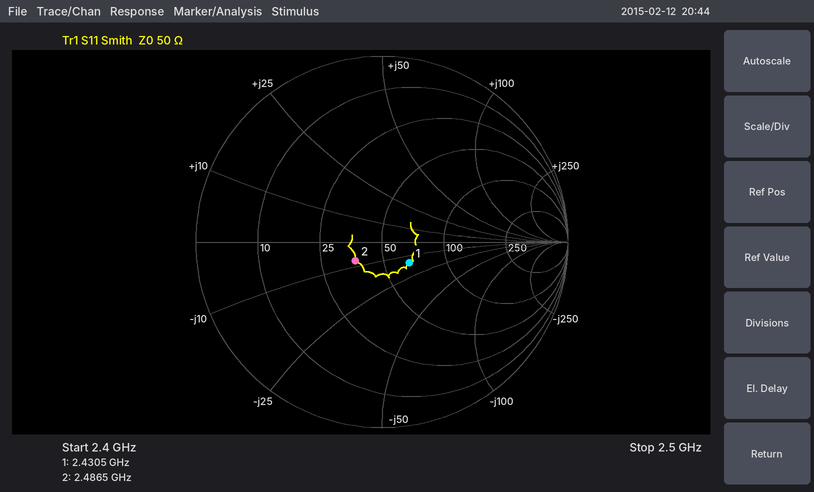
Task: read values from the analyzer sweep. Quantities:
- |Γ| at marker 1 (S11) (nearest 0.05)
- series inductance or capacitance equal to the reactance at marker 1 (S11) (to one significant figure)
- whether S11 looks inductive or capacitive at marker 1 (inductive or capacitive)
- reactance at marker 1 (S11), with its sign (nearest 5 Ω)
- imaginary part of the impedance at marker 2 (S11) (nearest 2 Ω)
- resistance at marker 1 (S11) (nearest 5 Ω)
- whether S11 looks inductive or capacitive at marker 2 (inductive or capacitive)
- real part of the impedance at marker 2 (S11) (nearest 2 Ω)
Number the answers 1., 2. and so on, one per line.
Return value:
1. 0.20
2. 4 pF
3. capacitive
4. -15 Ω
5. -8 Ω
6. 65 Ω
7. capacitive
8. 36 Ω
